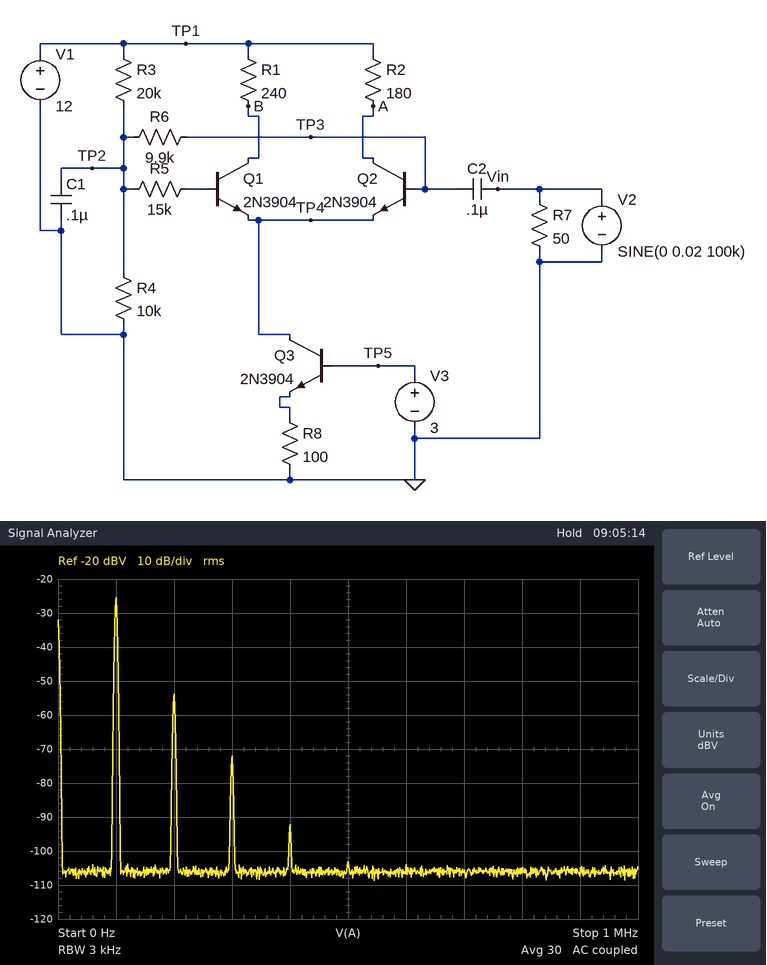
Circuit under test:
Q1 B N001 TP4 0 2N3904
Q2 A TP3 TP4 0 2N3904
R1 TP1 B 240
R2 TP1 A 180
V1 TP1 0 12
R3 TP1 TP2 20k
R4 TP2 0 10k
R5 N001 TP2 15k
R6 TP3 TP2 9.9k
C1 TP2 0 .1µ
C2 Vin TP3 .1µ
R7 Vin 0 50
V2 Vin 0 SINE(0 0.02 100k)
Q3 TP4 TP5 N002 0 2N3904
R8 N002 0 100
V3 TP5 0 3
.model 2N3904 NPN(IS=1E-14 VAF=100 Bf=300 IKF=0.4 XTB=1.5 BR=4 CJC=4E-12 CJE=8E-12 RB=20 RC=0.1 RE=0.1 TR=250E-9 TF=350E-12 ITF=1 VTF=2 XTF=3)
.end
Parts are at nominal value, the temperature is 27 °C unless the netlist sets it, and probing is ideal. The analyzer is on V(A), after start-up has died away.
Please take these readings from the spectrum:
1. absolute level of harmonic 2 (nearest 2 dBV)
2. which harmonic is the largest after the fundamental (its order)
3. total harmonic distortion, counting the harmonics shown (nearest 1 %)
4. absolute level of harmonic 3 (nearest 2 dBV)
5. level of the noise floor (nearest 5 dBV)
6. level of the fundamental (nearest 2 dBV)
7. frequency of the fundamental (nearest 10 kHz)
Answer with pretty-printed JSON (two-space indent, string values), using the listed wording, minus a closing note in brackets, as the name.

{
  "absolute level of harmonic 2": "-54 dBV",
  "which harmonic is the largest after the fundamental": "2",
  "total harmonic distortion, counting the harmonics shown": "4 %",
  "absolute level of harmonic 3": "-72 dBV",
  "level of the noise floor": "-105 dBV",
  "level of the fundamental": "-26 dBV",
  "frequency of the fundamental": "100 kHz"
}
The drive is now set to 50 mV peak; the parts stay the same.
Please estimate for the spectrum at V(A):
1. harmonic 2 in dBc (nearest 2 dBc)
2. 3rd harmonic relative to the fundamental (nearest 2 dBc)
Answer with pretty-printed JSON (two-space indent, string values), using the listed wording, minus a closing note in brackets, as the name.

{
  "harmonic 2 in dBc": "-20 dBc",
  "3rd harmonic relative to the fundamental": "-32 dBc"
}
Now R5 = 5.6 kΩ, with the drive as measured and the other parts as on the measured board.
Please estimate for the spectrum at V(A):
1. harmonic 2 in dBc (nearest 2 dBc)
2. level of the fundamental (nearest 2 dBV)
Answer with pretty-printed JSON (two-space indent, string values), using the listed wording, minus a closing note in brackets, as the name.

{
  "harmonic 2 in dBc": "-50 dBc",
  "level of the fundamental": "-20 dBV"
}
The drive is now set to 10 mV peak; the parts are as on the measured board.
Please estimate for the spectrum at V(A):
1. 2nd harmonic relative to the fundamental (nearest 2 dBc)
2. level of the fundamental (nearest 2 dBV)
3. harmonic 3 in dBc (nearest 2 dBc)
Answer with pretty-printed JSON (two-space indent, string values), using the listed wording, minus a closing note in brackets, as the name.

{
  "2nd harmonic relative to the fundamental": "-34 dBc",
  "level of the fundamental": "-32 dBV",
  "harmonic 3 in dBc": "-58 dBc"
}
